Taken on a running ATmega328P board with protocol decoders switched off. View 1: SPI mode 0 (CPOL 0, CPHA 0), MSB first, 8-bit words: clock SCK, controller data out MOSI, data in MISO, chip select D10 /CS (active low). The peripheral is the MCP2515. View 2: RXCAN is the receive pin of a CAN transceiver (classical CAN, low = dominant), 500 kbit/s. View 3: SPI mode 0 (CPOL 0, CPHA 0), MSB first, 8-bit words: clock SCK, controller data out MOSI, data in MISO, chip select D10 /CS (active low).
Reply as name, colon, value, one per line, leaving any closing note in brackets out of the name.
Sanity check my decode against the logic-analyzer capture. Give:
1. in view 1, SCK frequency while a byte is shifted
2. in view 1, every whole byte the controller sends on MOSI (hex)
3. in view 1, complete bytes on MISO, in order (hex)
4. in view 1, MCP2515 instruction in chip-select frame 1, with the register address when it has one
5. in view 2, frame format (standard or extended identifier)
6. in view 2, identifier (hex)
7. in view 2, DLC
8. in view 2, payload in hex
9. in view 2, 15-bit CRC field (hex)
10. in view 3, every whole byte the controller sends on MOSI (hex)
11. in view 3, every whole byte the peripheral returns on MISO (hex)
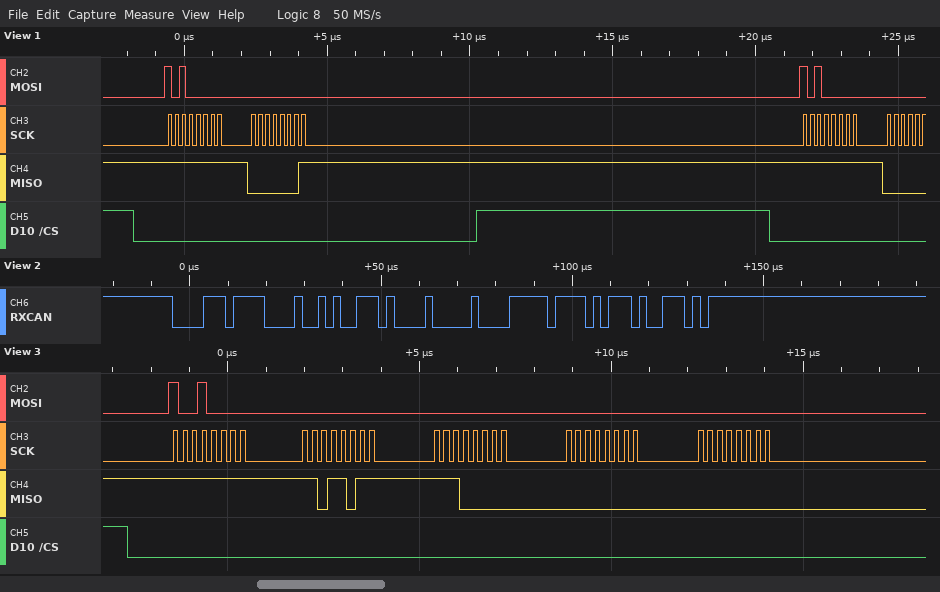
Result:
in view 1, SCK frequency while a byte is shifted: 4 MHz
in view 1, every whole byte the controller sends on MOSI: 0xA0 0x00 0xA0
in view 1, complete bytes on MISO, in order: 0xFF 0x01 0xFF
in view 1, MCP2515 instruction in chip-select frame 1, with the register address when it has one: READ STATUS
in view 2, frame format: standard
in view 2, identifier: 0x0EF
in view 2, DLC: 4
in view 2, payload in hex: A7 42 00 FF
in view 2, 15-bit CRC field: 0x574E
in view 3, every whole byte the controller sends on MOSI: 90 00 00 00 00
in view 3, every whole byte the peripheral returns on MISO: FF DB E0 00 00
